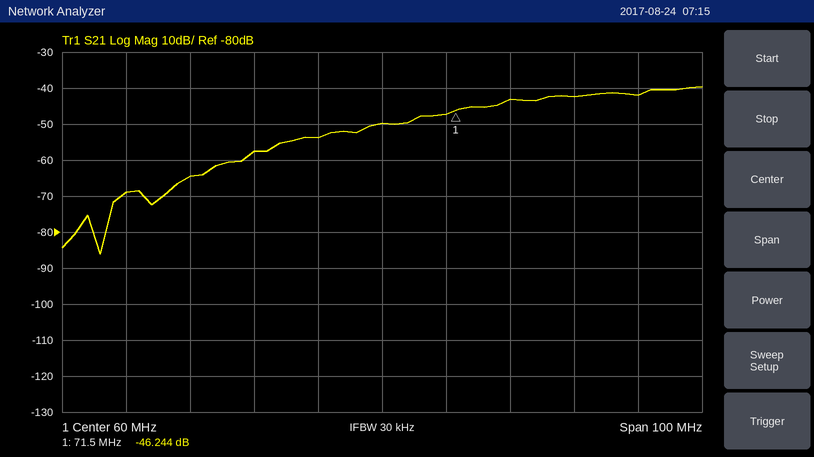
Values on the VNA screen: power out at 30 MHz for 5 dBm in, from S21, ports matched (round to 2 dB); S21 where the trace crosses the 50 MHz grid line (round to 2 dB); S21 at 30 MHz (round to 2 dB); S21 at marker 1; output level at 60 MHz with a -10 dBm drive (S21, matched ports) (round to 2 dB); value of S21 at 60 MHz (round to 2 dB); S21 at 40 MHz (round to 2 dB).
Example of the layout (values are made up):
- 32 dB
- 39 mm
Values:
- -60 dBm
- -54 dB
- -64 dB
- -46.244 dB
- -60 dBm
- -50 dB
- -58 dB
